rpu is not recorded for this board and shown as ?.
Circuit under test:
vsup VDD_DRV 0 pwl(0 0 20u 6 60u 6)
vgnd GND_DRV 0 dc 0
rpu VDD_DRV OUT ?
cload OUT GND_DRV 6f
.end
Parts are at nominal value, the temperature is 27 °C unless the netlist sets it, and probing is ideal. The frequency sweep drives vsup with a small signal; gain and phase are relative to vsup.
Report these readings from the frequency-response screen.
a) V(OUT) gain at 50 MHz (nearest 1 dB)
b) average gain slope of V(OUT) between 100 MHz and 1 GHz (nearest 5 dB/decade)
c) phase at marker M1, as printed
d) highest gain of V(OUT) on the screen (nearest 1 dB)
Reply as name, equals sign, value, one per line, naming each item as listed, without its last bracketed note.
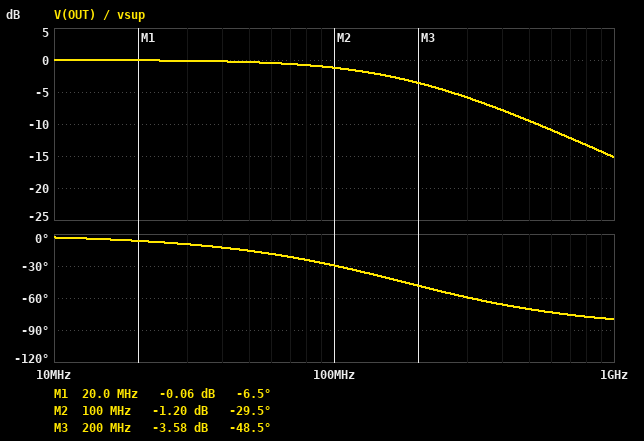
V(OUT) gain at 50 MHz = 0 dB
average gain slope of V(OUT) between 100 MHz and 1 GHz = -15 dB/decade
phase at marker M1, as printed = -6.5 deg
highest gain of V(OUT) on the screen = 0 dB
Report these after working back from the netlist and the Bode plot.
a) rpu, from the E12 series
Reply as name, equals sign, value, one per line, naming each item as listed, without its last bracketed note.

rpu, from the E12 series = 150 kΩ
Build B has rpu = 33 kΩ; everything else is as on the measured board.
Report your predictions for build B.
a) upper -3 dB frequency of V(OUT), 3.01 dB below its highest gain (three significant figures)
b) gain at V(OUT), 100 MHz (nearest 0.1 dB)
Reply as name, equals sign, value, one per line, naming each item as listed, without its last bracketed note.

upper -3 dB frequency of V(OUT), 3.01 dB below its highest gain = 804 MHz
gain at V(OUT), 100 MHz = -0.1 dB
